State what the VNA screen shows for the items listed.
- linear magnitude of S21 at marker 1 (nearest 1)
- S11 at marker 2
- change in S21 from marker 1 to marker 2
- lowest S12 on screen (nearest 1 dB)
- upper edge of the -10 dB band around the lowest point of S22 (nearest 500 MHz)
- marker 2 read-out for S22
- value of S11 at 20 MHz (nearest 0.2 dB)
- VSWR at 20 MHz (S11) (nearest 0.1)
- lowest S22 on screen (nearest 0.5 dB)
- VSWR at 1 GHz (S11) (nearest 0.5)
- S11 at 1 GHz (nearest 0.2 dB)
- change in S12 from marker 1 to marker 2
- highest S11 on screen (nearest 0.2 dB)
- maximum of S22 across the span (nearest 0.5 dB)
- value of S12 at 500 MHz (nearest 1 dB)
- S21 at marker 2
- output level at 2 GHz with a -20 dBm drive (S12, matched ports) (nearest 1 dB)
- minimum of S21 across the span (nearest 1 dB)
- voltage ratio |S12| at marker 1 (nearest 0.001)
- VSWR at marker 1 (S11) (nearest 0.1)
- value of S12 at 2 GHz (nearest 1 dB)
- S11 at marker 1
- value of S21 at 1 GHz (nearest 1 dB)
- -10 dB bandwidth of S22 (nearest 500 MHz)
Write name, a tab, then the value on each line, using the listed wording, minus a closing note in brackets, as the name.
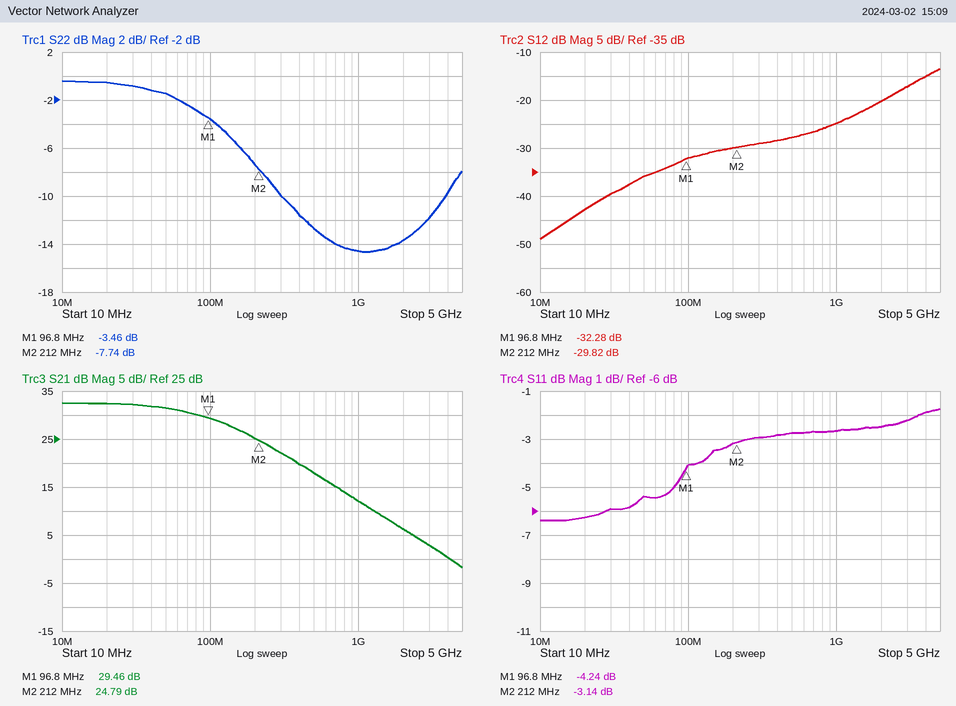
linear magnitude of S21 at marker 1	30
S11 at marker 2	-3.14 dB
change in S21 from marker 1 to marker 2	-4.67 dB
lowest S12 on screen	-49 dB
upper edge of the -10 dB band around the lowest point of S22	4.0 GHz
marker 2 read-out for S22	-7.74 dB
value of S11 at 20 MHz	-6.2 dB
VSWR at 20 MHz (S11)	2.9
lowest S22 on screen	-14.5 dB
VSWR at 1 GHz (S11)	6.5
S11 at 1 GHz	-2.6 dB
change in S12 from marker 1 to marker 2	2.46 dB
highest S11 on screen	-1.8 dB
maximum of S22 across the span	-0.5 dB
value of S12 at 500 MHz	-28 dB
S21 at marker 2	24.79 dB
output level at 2 GHz with a -20 dBm drive (S12, matched ports)	-40 dBm
minimum of S21 across the span	-2 dB
voltage ratio |S12| at marker 1	0.024
VSWR at marker 1 (S11)	4.2
value of S12 at 2 GHz	-20 dB
S11 at marker 1	-4.24 dB
value of S21 at 1 GHz	12 dB
-10 dB bandwidth of S22	3.5 GHz
